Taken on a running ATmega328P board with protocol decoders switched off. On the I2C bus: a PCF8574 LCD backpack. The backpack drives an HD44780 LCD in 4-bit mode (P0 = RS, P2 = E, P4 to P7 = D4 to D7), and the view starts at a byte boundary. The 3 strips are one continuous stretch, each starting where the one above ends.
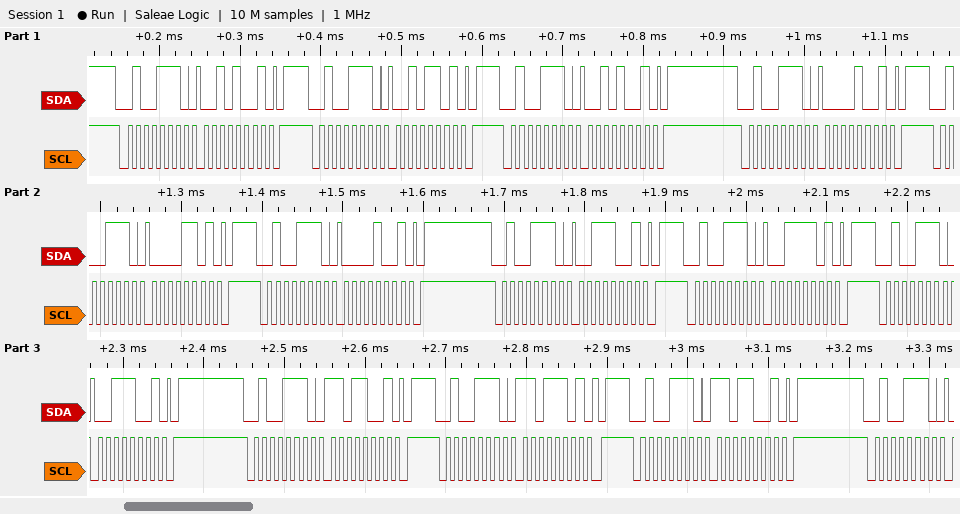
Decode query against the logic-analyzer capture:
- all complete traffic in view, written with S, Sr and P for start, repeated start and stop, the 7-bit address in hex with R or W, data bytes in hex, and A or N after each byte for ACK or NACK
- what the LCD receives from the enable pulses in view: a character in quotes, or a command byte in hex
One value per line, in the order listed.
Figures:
S 27W A 29 A P S 27W A 2D A P S 27W A 29 A P S 27W A 09 A P S 27W A 0D A P S 27W A 09 A P S 27W A 39 A P S 27W A 3D A P S 27W A 39 A P S 27W A D9 A P S 27W A DD A P S 27W A D9 A P S 27W A
' ' '='
